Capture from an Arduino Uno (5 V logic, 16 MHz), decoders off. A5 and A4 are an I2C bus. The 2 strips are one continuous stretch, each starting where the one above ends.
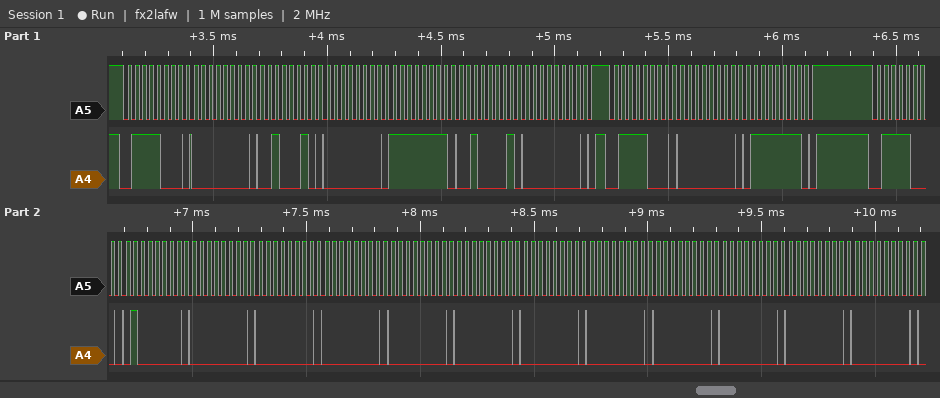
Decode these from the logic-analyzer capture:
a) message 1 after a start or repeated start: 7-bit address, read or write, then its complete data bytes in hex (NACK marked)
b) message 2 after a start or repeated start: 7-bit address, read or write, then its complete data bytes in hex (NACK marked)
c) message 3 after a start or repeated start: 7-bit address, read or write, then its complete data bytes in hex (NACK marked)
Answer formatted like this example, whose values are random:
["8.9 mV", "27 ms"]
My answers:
["0x3C write: 00 22 00 FF 21 00", "0x3C write: 00 7F", "0x3C write: 40 00 00 00 00 00 00 00 00 00 00 00"]
